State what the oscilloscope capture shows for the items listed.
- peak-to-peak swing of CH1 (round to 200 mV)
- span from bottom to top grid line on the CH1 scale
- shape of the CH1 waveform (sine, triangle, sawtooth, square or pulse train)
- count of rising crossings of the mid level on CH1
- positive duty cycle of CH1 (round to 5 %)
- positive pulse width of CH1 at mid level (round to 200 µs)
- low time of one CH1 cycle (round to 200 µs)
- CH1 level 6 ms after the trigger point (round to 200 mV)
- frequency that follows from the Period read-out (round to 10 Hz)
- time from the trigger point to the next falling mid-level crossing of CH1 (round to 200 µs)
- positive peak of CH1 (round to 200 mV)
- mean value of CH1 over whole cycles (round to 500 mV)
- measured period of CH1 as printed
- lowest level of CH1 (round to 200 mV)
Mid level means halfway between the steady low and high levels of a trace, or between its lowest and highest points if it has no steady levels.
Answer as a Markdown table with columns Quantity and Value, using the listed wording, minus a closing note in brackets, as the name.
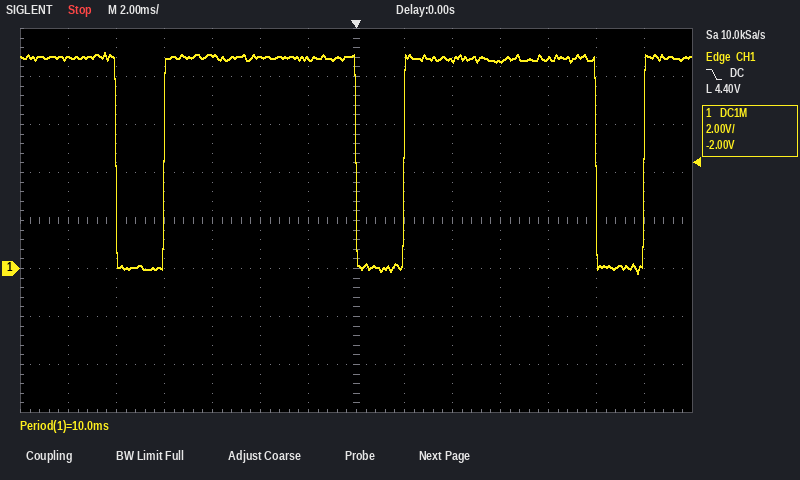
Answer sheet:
| Quantity | Value |
|---|---|
| peak-to-peak swing of CH1 | 9.2 V |
| span from bottom to top grid line on the CH1 scale | 16 V |
| shape of the CH1 waveform | pulse train |
| count of rising crossings of the mid level on CH1 | 3 |
| positive duty cycle of CH1 | 80 % |
| positive pulse width of CH1 at mid level | 8.0 ms |
| low time of one CH1 cycle | 2.0 ms |
| CH1 level 6 ms after the trigger point | 8.6 V |
| frequency that follows from the Period read-out | 100 Hz |
| time from the trigger point to the next falling mid-level crossing of CH1 | 10.0 ms |
| positive peak of CH1 | 9.0 V |
| mean value of CH1 over whole cycles | 7.0 V |
| measured period of CH1 as printed | 10.0 ms |
| lowest level of CH1 | -200 mV |
